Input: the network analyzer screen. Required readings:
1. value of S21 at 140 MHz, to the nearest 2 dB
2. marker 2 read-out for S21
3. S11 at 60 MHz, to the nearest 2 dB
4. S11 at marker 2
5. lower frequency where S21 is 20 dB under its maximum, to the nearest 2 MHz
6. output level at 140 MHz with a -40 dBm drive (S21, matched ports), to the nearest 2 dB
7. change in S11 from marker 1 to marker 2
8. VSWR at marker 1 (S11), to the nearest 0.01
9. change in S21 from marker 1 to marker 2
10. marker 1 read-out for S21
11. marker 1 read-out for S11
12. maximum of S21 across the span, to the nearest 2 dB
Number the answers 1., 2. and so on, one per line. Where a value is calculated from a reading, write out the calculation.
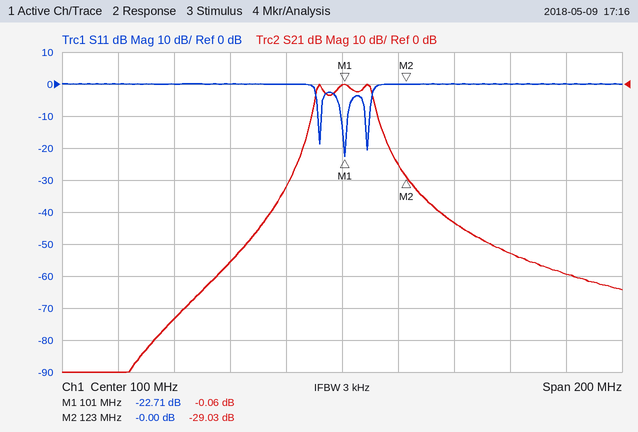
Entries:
1. -44 dB
2. -29.03 dB
3. 0 dB
4. -0.00 dB
5. 86 MHz
6. -40 dBm + (-44 dB) = -84 dBm
7. -0 − (-22.71) = 22.71 dB
8. (1 + 0.0732)/(1 − 0.0732) ≈ 1.16
9. -29.03 − (-0.06) = -28.97 dB
10. -0.06 dB
11. -22.71 dB
12. 0 dB
